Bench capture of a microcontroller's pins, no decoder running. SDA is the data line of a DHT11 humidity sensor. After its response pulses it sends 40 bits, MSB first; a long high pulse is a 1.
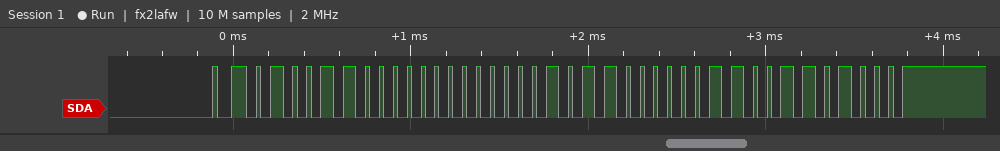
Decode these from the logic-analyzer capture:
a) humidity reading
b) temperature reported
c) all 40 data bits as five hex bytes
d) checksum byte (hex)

76 %
22.6 °C
4C 00 16 06 68
0x68
